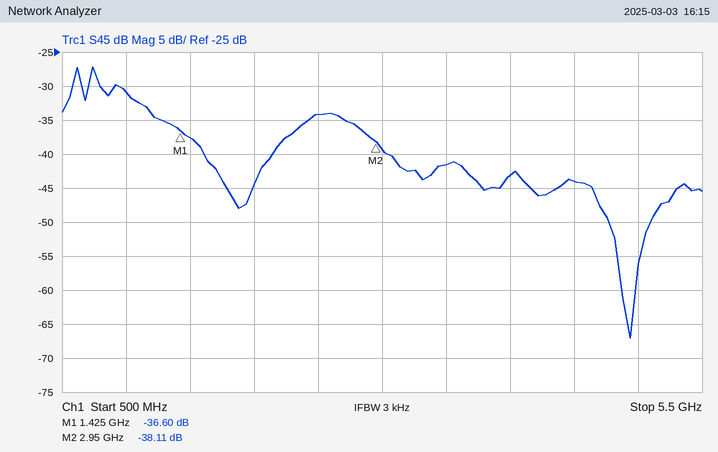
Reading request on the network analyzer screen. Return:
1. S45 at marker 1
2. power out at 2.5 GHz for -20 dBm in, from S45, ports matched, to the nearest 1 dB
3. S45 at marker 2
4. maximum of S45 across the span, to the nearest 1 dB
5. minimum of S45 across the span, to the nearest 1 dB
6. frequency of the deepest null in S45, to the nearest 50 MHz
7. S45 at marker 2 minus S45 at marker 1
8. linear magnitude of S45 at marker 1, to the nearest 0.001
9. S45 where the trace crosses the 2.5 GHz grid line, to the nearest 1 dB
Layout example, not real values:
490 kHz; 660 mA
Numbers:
-36.60 dB; -54 dBm; -38.11 dB; -27 dB; -67 dB; 4.95 GHz; -1.51 dB; 0.015; -34 dB
